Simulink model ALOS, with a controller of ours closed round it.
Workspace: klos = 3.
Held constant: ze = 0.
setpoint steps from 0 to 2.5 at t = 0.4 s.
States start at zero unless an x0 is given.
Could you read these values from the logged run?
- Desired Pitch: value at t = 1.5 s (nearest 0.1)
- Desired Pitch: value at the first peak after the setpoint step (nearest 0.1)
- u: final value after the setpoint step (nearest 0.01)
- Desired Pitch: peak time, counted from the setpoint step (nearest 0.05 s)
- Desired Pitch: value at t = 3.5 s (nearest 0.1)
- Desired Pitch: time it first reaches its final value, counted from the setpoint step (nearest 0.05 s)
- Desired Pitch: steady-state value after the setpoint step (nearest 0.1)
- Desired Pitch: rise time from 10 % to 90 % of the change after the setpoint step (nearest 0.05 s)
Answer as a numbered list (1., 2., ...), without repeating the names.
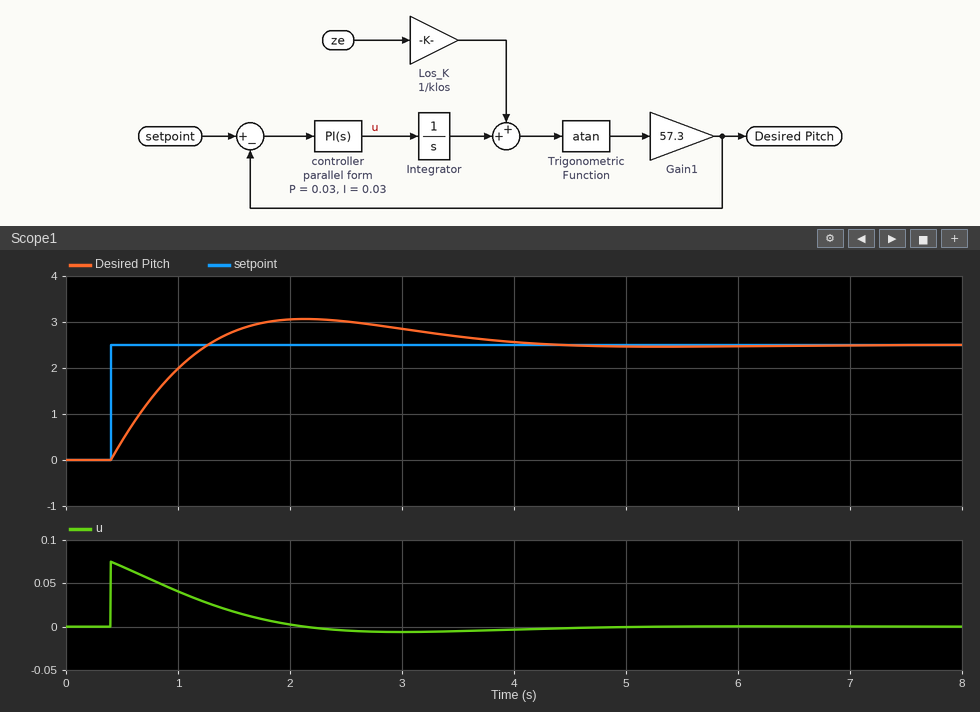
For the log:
1. 2.8
2. 3.1
3. 0.00
4. 1.75 s
5. 2.7
6. 0.85 s
7. 2.5
8. 0.65 s
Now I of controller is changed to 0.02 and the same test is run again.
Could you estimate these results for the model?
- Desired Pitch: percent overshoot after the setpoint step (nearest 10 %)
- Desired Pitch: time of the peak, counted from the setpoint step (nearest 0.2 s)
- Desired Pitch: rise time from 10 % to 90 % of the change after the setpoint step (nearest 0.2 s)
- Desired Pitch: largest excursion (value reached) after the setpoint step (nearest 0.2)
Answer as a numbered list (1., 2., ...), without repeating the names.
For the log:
1. 20 %
2. 2.0 s
3. 0.8 s
4. 3.0
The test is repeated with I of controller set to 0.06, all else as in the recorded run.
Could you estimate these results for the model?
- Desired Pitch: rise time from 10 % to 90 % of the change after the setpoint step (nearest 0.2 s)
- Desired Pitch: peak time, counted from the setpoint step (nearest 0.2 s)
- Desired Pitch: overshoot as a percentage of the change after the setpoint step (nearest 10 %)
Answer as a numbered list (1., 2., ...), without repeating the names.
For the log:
1. 0.6 s
2. 1.4 s
3. 30 %
